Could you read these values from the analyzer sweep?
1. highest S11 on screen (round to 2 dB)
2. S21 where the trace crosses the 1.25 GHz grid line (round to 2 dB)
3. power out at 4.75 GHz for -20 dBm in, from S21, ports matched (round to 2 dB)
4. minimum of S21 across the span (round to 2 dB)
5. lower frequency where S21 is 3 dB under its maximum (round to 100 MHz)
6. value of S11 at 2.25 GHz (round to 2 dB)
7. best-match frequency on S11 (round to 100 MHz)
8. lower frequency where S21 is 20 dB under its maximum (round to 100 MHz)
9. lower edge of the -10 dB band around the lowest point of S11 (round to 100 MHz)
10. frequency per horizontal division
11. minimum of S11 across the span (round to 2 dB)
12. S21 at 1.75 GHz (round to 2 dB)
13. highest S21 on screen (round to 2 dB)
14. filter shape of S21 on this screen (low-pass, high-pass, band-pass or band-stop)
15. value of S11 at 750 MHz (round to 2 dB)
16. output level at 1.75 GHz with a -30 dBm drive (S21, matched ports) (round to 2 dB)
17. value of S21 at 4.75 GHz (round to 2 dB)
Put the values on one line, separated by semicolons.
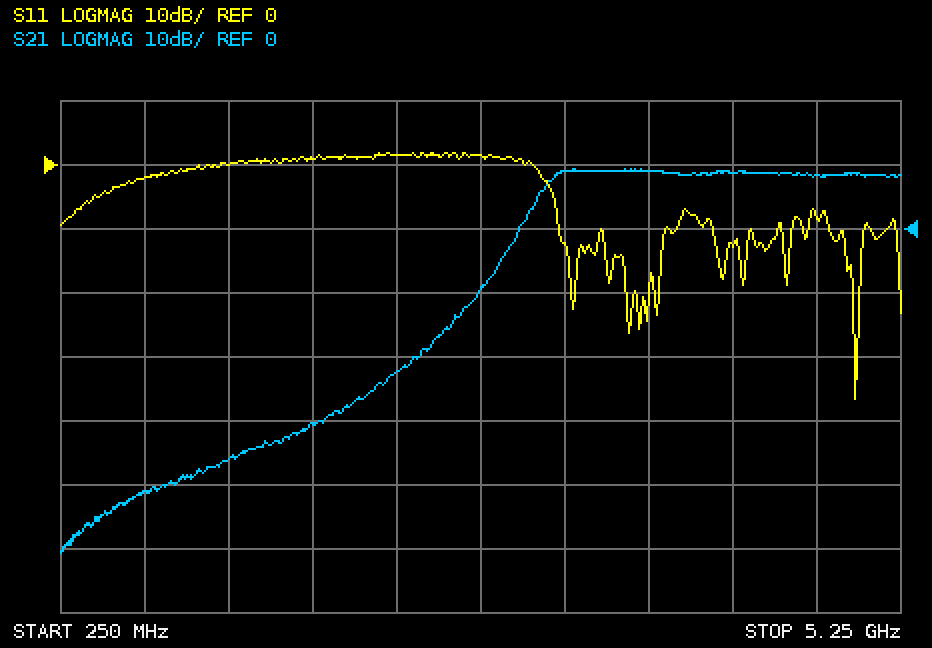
2 dB; -36 dB; -12 dBm; -50 dB; 3.1 GHz; 2 dB; 5.0 GHz; 2.7 GHz; 4.8 GHz; 500 MHz; -36 dB; -30 dB; 10 dB; high-pass; -2 dB; -60 dBm; 8 dB
